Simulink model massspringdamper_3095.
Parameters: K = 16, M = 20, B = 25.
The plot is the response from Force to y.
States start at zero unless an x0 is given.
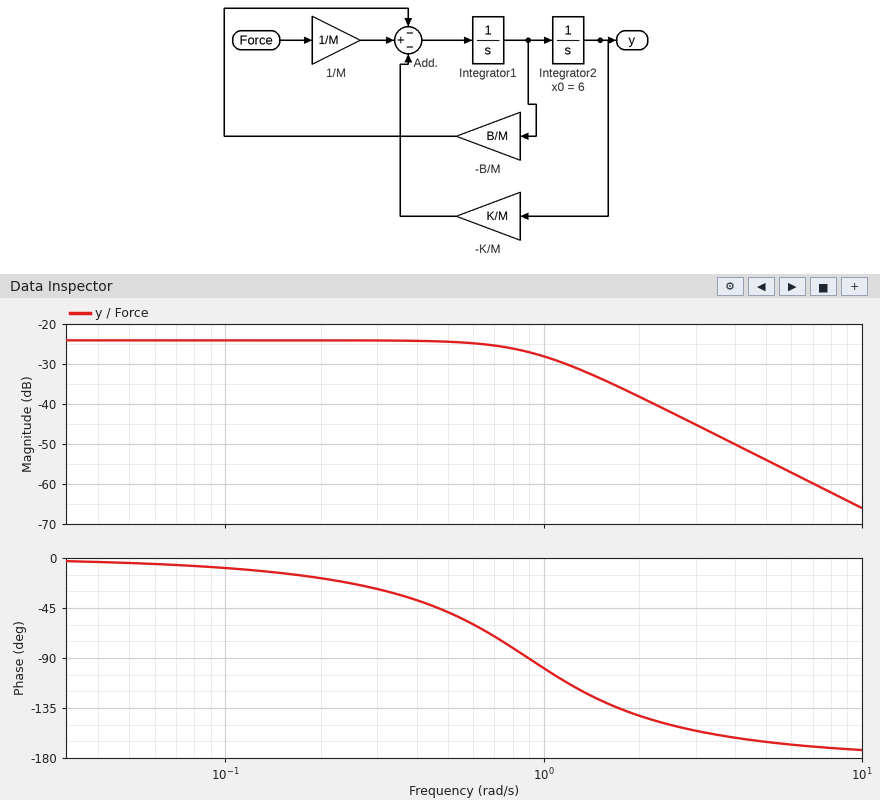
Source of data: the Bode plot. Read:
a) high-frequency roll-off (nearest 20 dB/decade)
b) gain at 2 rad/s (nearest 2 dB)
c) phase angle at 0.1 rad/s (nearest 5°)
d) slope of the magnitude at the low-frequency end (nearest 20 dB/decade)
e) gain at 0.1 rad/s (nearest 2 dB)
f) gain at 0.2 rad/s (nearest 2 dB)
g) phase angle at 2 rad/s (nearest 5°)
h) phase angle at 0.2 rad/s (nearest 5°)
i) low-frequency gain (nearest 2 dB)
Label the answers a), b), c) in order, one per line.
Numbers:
a) -40 dB/decade
b) -38 dB
c) -10°
d) 0 dB/decade
e) -24 dB
f) -24 dB
g) -140°
h) -20°
i) -24 dB
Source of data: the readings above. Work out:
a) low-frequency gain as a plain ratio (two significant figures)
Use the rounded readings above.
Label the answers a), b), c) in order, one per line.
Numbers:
a) 0.063
